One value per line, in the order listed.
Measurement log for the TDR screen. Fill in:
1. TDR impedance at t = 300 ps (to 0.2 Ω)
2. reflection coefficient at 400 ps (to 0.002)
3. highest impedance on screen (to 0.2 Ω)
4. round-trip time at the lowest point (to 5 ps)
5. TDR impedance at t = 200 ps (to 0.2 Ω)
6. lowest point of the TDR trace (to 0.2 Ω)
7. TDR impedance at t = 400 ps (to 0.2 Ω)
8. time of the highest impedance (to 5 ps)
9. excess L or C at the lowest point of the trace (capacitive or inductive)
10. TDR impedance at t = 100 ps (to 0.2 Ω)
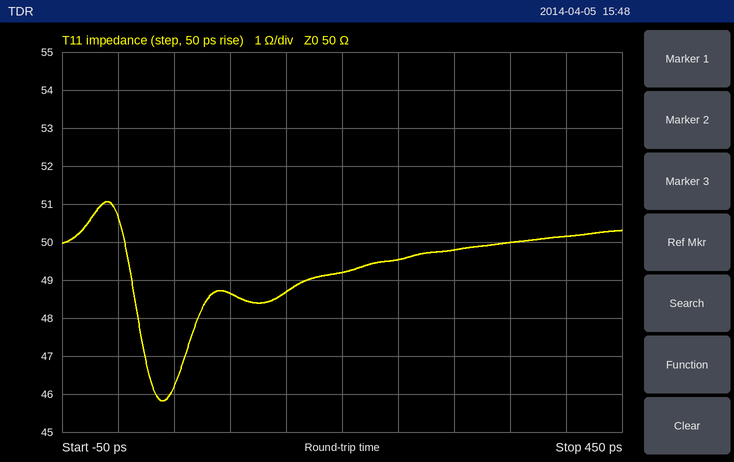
49.8 Ω
+0.002
51.0 Ω
40 ps
49.2 Ω
45.8 Ω
50.2 Ω
-10 ps
capacitive
48.6 Ω
